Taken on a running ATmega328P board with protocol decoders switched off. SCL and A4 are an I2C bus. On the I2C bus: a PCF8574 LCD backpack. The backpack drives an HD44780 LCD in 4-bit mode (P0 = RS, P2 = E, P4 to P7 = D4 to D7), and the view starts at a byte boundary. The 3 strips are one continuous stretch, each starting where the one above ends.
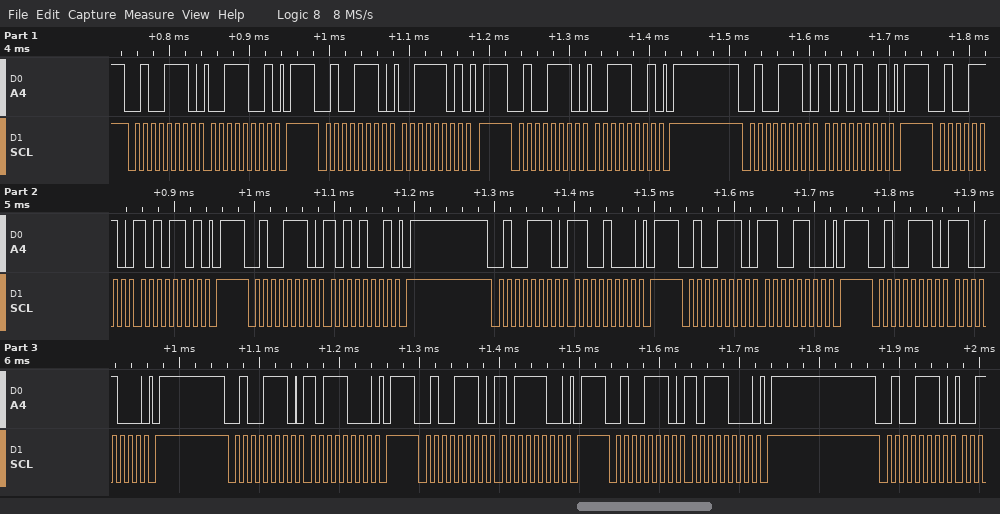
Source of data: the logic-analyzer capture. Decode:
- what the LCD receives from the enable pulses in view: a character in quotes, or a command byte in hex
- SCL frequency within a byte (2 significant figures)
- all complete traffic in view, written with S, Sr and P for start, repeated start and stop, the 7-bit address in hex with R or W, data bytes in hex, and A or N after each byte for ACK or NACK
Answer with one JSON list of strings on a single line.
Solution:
["':' 0xCB", "100 kHz", "S 27W A 39 A P S 27W A 3D A P S 27W A 39 A P S 27W A A9 A P S 27W A AD A P S 27W A A9 A P S 27W A C8 A P S 27W A CC A P S 27W A C8 A P S 27W A B8 A P S 27W A BC A P S 27W A B8 A P S 27W A"]
